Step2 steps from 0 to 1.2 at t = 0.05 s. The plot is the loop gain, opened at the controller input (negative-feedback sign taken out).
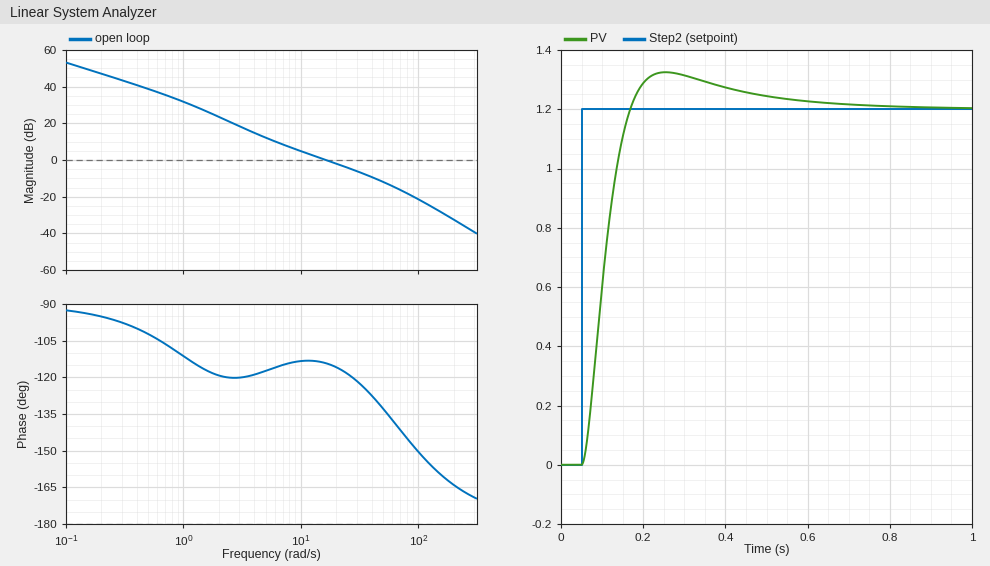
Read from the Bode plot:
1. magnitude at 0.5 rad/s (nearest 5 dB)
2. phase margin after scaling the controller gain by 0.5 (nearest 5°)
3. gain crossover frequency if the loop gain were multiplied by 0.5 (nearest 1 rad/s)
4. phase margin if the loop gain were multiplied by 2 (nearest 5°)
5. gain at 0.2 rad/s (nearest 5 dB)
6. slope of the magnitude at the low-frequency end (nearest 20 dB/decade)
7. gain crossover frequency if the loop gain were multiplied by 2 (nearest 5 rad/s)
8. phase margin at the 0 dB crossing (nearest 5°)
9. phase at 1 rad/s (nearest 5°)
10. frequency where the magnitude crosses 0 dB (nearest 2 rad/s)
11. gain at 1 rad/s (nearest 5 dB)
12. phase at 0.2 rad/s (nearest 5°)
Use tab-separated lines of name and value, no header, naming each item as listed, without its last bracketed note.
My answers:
magnitude at 0.5 rad/s	40 dB
phase margin after scaling the controller gain by 0.5	65°
gain crossover frequency if the loop gain were multiplied by 0.5	9 rad/s
phase margin if the loop gain were multiplied by 2	60°
gain at 0.2 rad/s	45 dB
slope of the magnitude at the low-frequency end	-20 dB/decade
gain crossover frequency if the loop gain were multiplied by 2	30 rad/s
phase margin at the 0 dB crossing	65°
phase at 1 rad/s	-110°
frequency where the magnitude crosses 0 dB	16 rad/s
gain at 1 rad/s	30 dB
phase at 0.2 rad/s	-95°
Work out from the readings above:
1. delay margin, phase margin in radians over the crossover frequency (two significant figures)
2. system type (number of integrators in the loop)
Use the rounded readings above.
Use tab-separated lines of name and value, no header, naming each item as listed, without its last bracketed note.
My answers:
delay margin, phase margin in radians over the crossover frequency	0.071 s
system type	1
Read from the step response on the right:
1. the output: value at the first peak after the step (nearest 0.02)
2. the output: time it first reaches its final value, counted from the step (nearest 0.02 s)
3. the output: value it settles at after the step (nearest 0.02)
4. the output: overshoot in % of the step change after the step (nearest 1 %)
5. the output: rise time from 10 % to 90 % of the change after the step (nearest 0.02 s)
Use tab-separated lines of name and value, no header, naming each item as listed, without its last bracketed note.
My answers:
the output: value at the first peak after the step	1.32
the output: time it first reaches its final value, counted from the step	0.12 s
the output: value it settles at after the step	1.20
the output: overshoot in % of the step change after the step	10 %
the output: rise time from 10 % to 90 % of the change after the step	0.08 s
